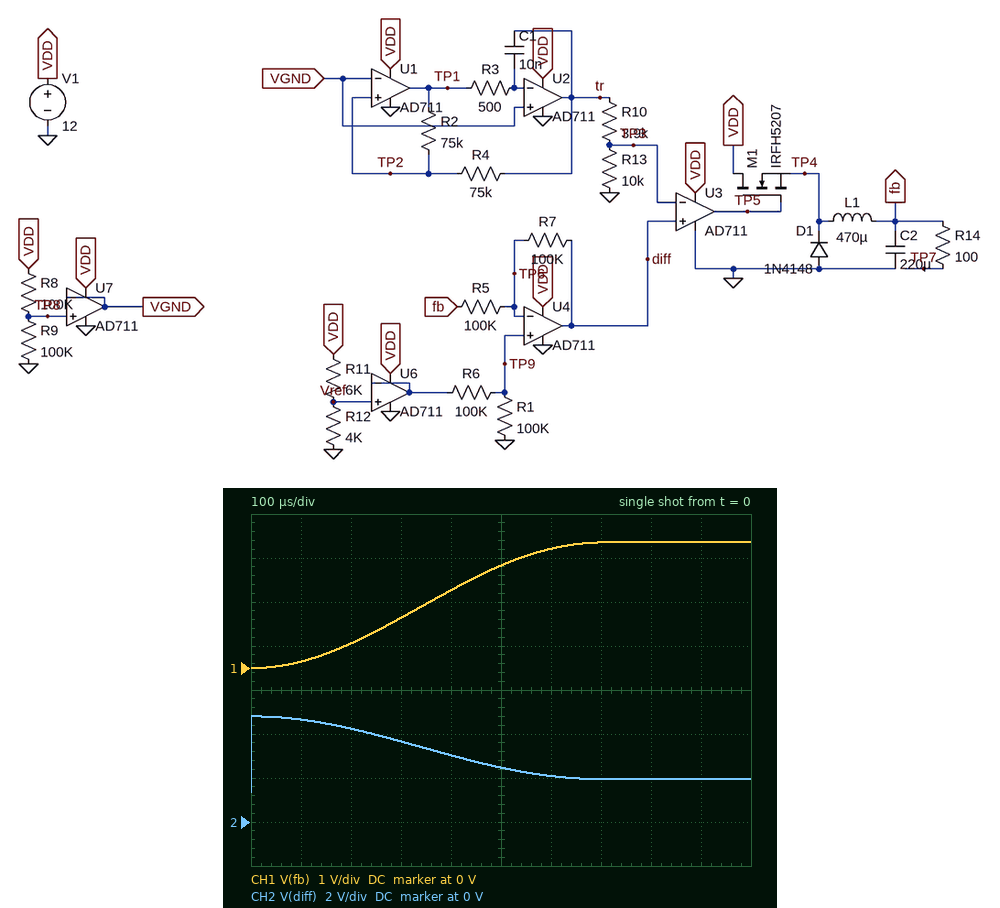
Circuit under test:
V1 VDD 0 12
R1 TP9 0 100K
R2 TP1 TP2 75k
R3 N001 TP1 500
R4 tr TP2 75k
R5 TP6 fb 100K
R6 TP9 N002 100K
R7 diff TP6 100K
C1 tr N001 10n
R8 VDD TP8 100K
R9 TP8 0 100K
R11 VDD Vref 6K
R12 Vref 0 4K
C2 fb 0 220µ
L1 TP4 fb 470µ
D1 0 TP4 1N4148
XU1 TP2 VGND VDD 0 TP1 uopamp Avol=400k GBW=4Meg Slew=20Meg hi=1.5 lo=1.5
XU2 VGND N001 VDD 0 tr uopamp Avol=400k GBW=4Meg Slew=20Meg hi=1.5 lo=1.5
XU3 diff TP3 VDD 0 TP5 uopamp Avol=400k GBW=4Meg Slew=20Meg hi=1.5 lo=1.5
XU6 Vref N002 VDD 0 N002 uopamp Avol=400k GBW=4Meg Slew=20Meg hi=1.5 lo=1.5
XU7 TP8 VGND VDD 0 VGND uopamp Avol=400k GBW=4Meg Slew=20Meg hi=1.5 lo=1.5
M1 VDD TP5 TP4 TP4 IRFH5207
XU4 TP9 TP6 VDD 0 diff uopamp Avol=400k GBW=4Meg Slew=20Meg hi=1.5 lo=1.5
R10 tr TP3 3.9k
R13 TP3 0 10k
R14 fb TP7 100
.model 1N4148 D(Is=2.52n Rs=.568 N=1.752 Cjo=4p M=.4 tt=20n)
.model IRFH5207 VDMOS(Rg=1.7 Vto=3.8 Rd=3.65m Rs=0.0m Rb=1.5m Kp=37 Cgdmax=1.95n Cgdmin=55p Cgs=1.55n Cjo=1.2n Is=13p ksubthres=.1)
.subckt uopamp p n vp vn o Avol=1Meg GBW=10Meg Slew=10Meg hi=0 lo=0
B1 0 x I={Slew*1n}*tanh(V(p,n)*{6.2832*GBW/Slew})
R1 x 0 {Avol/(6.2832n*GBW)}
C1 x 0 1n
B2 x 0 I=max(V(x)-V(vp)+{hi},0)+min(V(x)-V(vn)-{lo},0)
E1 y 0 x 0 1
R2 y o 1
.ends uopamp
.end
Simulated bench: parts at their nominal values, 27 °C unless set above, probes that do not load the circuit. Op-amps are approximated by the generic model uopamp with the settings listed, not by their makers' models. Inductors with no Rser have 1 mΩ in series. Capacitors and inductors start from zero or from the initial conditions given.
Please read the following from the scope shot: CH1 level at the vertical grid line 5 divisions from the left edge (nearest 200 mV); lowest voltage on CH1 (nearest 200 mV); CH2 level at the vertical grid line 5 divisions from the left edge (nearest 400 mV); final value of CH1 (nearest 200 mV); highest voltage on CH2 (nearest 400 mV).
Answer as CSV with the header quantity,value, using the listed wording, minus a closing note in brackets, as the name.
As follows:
quantity,value
CH1 level at the vertical grid line 5 divisions from the left edge,2.4 V
lowest voltage on CH1,0 V
CH2 level at the vertical grid line 5 divisions from the left edge,2.4 V
final value of CH1,2.8 V
highest voltage on CH2,4.8 V
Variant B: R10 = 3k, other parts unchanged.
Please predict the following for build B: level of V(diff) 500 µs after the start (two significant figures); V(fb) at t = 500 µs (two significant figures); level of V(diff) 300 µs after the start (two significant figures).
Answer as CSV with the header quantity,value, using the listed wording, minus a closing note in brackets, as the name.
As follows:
quantity,value
level of V(diff) 500 µs after the start,2.7 V
V(fb) at t = 500 µs,2.1 V
level of V(diff) 300 µs after the start,3.8 V
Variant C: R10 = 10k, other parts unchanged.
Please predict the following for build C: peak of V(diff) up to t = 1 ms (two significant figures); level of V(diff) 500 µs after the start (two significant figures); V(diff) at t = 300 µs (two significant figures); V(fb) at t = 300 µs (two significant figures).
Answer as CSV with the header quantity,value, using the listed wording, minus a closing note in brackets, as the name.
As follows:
quantity,value
peak of V(diff) up to t = 1 ms,4.8 V
level of V(diff) 500 µs after the start,1.5 V
V(diff) at t = 300 µs,2.9 V
V(fb) at t = 300 µs,1.9 V
